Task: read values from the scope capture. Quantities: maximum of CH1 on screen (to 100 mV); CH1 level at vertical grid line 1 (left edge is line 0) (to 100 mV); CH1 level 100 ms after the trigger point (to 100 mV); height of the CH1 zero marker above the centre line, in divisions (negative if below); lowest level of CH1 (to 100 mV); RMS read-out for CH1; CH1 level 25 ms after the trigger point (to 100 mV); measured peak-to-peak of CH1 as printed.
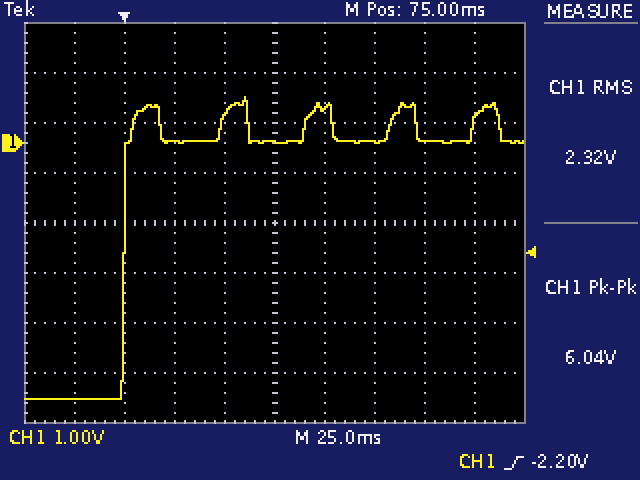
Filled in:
900 mV
-5.1 V
700 mV
+1.6 div
-5.1 V
2.32 V
0.0 V
6.04 V
